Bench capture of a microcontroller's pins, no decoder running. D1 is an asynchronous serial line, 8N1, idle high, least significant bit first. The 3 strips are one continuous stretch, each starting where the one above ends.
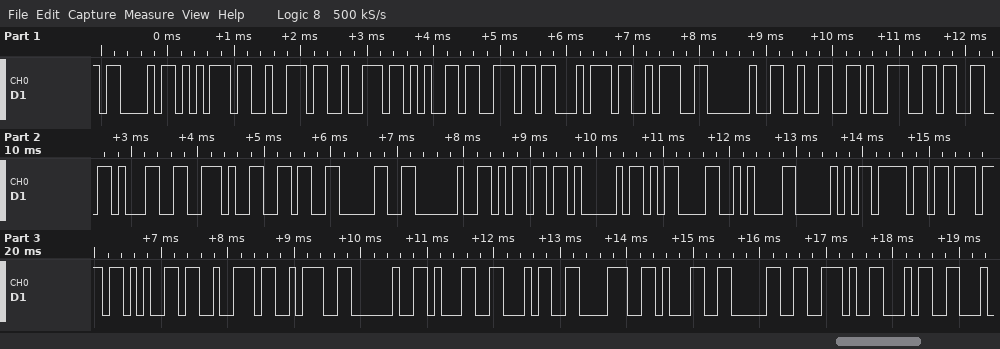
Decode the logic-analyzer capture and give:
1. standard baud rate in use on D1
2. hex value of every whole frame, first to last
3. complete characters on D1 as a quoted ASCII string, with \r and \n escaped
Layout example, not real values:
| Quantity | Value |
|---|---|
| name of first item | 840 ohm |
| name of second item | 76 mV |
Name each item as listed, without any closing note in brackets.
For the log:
| Quantity | Value |
|---|---|
| standard baud rate in use on D1 | 9600 baud |
| hex value of every whole frame, first to last | 43 75 72 72 65 6E 74 3A 20 32 39 33 31 2E 36 30 20 6D 41 0D 0A 50 6F 77 65 72 3A 20 31 34 38 31 30 2E 34 |
| complete characters on D1 as a quoted ASCII string, with \r and \n escaped | "Current: 2931.60 mA\r\nPower: 14810.4" |
